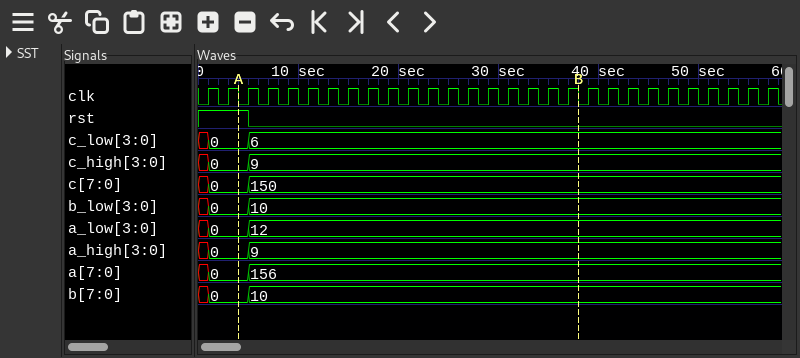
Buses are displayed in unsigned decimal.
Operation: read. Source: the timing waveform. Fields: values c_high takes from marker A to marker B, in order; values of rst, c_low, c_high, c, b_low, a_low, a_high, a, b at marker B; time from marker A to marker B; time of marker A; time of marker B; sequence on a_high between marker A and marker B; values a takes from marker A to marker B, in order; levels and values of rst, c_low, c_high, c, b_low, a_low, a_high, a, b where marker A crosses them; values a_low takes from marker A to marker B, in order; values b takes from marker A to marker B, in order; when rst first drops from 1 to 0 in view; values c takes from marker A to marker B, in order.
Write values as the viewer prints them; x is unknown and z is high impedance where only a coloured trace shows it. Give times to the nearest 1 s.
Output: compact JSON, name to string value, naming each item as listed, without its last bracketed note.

{"values c_high takes from marker A to marker B, in order": "0, 9", "values of rst, c_low, c_high, c, b_low, a_low, a_high, a, b at marker B": "rst=0, c_low=6, c_high=9, c=150, b_low=10, a_low=12, a_high=9, a=156, b=10", "time from marker A to marker B": "34 s", "time of marker A": "4 s", "time of marker B": "38 s", "sequence on a_high between marker A and marker B": "0, 9", "values a takes from marker A to marker B, in order": "0, 156", "levels and values of rst, c_low, c_high, c, b_low, a_low, a_high, a, b where marker A crosses them": "rst=1, c_low=0, c_high=0, c=0, b_low=0, a_low=0, a_high=0, a=0, b=0", "values a_low takes from marker A to marker B, in order": "0, 12", "values b takes from marker A to marker B, in order": "0, 10", "when rst first drops from 1 to 0 in view": "5 s", "values c takes from marker A to marker B, in order": "0, 150"}
